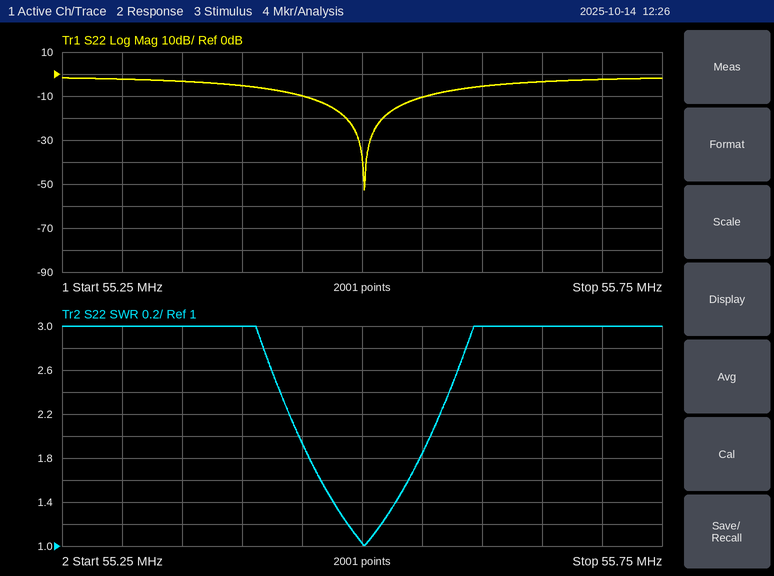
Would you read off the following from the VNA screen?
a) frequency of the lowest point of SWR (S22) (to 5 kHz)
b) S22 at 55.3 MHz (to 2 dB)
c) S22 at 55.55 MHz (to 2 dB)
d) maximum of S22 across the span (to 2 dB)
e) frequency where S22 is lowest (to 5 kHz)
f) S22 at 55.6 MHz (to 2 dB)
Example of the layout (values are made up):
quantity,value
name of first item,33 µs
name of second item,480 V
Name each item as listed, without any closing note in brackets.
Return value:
quantity,value
frequency of the lowest point of SWR (S22),55.500 MHz
S22 at 55.3 MHz,-2 dB
S22 at 55.55 MHz,-10 dB
maximum of S22 across the span,-2 dB
frequency where S22 is lowest,55.500 MHz
S22 at 55.6 MHz,-6 dB
